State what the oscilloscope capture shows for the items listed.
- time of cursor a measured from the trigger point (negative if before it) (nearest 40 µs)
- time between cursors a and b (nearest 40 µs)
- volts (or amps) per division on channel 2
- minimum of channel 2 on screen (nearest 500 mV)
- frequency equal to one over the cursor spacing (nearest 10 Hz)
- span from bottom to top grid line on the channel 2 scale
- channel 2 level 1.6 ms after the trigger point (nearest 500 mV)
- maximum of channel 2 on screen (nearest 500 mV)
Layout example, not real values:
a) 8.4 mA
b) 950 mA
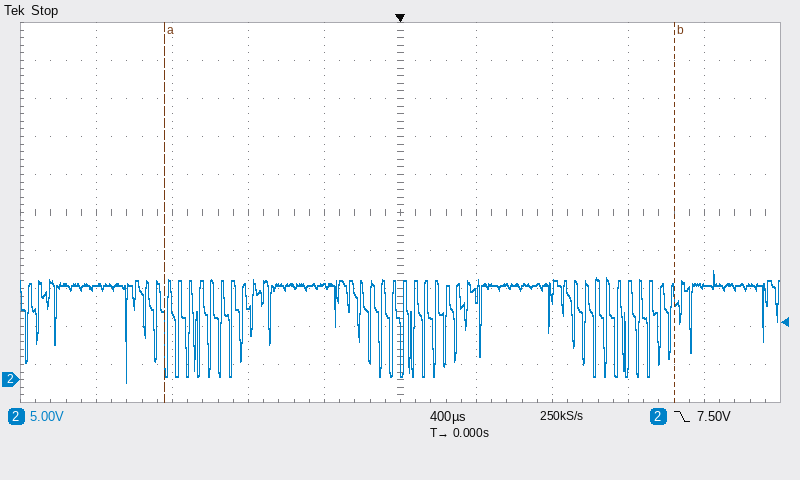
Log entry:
a) -1.24 ms
b) 2.68 ms
c) 5 V
d) -500 mV
e) 370 Hz
f) 50 V
g) 12.5 V
h) 14.5 V
